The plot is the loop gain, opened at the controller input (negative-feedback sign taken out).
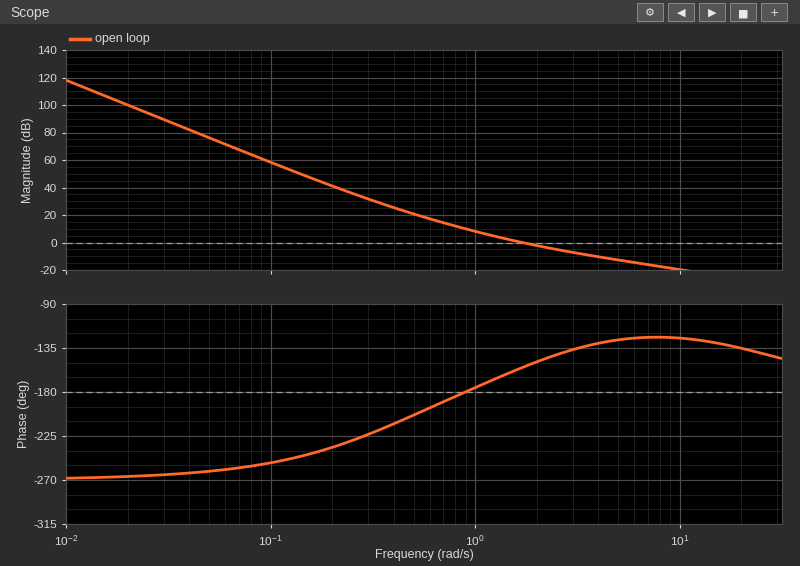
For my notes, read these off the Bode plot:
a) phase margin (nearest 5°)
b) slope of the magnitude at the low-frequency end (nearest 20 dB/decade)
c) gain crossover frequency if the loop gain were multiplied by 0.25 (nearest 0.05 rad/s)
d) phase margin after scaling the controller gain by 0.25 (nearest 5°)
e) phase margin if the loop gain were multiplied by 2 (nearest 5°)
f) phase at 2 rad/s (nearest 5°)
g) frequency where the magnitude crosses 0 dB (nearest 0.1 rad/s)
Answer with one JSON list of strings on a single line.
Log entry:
["25°", "-60 dB/decade", "0.80 rad/s", "-5°", "40°", "-150°", "1.7 rad/s"]
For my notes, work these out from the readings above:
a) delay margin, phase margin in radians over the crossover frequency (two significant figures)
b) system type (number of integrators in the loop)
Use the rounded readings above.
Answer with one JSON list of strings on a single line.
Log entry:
["0.26 s", "3"]
